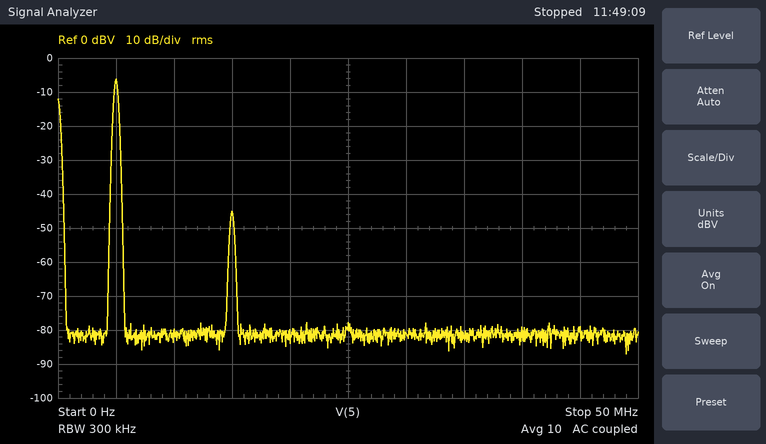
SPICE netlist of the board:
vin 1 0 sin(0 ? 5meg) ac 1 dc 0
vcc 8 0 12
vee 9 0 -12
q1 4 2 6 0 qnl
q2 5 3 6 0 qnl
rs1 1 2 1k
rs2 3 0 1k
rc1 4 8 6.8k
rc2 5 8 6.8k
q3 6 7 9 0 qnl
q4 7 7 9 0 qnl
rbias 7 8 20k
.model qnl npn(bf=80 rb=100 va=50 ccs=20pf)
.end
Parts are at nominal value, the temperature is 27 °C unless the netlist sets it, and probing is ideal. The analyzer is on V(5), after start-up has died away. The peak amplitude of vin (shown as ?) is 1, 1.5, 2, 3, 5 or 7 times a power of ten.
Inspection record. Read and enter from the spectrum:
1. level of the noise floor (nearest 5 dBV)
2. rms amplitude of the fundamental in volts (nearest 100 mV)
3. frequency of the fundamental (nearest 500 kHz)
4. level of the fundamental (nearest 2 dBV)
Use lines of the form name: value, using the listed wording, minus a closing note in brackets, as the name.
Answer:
level of the noise floor: -80 dBV
rms amplitude of the fundamental in volts: 500 mV
frequency of the fundamental: 5.0 MHz
level of the fundamental: -6 dBV
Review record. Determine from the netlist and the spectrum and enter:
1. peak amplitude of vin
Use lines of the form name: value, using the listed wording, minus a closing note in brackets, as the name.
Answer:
peak amplitude of vin: 50 mV
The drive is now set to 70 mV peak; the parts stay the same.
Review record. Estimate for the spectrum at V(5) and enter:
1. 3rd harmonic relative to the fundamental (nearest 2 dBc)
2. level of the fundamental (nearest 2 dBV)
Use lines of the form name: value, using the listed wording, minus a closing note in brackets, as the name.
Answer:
3rd harmonic relative to the fundamental: -34 dBc
level of the fundamental: -4 dBV
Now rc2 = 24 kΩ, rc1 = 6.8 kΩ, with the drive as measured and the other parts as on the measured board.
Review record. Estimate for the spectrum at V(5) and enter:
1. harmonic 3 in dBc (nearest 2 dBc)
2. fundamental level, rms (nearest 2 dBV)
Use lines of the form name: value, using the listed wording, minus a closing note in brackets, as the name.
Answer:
harmonic 3 in dBc: -22 dBc
fundamental level, rms: -10 dBV
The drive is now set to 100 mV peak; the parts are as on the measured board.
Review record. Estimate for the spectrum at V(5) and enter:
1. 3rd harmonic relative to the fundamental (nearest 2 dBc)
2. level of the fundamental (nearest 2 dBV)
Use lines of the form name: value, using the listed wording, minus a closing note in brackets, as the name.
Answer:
3rd harmonic relative to the fundamental: -28 dBc
level of the fundamental: -2 dBV
